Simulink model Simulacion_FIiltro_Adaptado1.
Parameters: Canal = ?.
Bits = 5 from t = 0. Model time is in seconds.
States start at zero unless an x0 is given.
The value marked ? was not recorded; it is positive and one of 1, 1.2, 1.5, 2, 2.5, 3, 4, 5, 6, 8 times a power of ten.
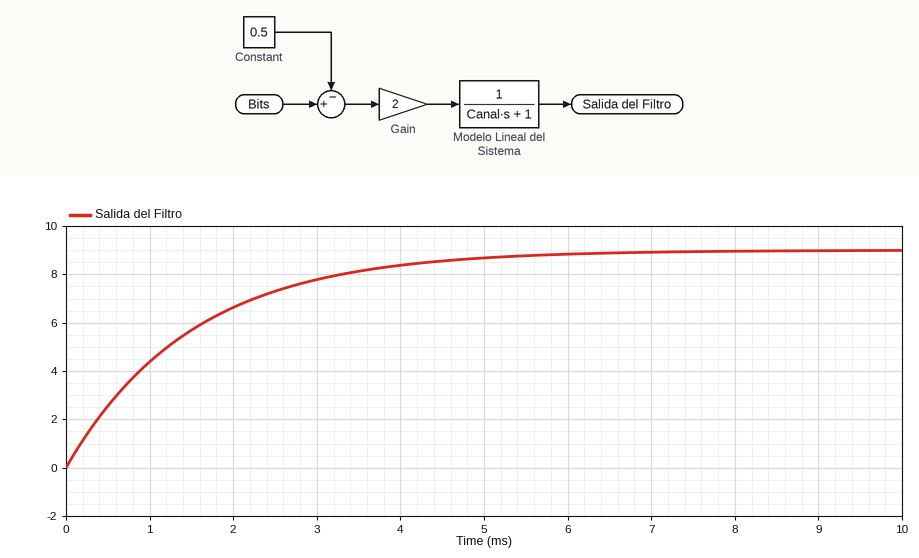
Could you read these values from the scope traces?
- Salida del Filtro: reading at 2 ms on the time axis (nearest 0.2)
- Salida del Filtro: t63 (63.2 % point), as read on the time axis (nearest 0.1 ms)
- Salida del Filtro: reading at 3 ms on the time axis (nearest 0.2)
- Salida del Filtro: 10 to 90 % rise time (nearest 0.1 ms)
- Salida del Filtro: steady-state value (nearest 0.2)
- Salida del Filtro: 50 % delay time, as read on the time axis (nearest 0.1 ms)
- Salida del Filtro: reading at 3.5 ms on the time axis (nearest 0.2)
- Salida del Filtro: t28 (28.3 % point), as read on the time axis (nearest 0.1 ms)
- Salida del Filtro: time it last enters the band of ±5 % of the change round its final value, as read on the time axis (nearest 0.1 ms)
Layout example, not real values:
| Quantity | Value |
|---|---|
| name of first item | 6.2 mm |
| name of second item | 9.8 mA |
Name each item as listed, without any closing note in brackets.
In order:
| Quantity | Value |
|---|---|
| Salida del Filtro: reading at 2 ms on the time axis | 6.6 |
| Salida del Filtro: t63 (63.2 % point), as read on the time axis | 1.5 ms |
| Salida del Filtro: reading at 3 ms on the time axis | 7.8 |
| Salida del Filtro: 10 to 90 % rise time | 3.3 ms |
| Salida del Filtro: steady-state value | 9.0 |
| Salida del Filtro: 50 % delay time, as read on the time axis | 1.0 ms |
| Salida del Filtro: reading at 3.5 ms on the time axis | 8.2 |
| Salida del Filtro: t28 (28.3 % point), as read on the time axis | 0.5 ms |
| Salida del Filtro: time it last enters the band of ±5 % of the change round its final value, as read on the time axis | 4.5 ms |
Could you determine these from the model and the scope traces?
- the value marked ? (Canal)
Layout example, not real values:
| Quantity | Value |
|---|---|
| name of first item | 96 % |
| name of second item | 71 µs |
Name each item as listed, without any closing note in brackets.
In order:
| Quantity | Value |
|---|---|
| the value marked ? | 0.0015 |
